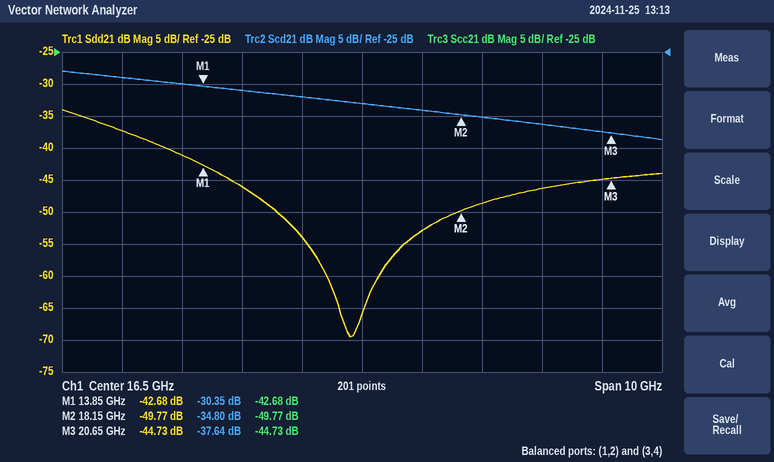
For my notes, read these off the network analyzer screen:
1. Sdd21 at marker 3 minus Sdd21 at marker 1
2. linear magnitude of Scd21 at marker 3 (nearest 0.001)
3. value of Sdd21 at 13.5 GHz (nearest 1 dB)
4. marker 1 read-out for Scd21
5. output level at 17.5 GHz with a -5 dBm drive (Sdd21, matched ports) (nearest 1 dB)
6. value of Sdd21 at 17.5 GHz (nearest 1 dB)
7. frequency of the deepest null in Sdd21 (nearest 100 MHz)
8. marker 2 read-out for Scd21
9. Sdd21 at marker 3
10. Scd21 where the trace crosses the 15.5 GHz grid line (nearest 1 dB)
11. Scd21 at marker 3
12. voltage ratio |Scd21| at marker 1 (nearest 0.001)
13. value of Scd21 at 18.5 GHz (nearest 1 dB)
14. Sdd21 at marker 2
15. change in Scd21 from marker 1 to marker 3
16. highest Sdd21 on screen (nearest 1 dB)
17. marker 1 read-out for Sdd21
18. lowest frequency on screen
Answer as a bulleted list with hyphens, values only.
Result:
- -2.05 dB
- 0.013
- -41 dB
- -30.35 dB
- -58 dBm
- -53 dB
- 16.3 GHz
- -34.80 dB
- -44.73 dB
- -32 dB
- -37.64 dB
- 0.030
- -35 dB
- -49.77 dB
- -7.29 dB
- -34 dB
- -42.68 dB
- 11.5 GHz
